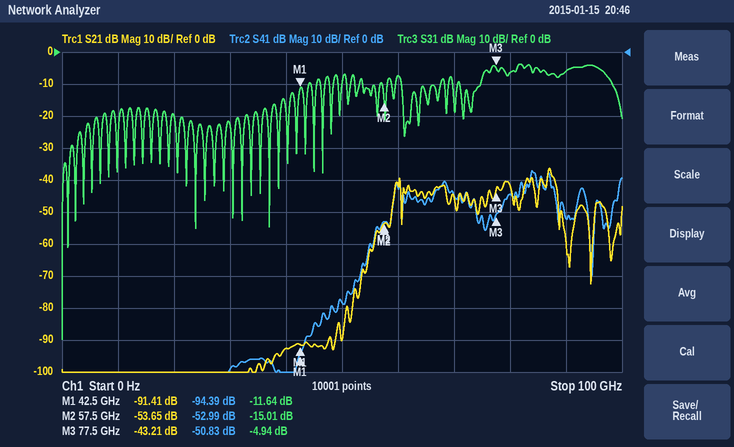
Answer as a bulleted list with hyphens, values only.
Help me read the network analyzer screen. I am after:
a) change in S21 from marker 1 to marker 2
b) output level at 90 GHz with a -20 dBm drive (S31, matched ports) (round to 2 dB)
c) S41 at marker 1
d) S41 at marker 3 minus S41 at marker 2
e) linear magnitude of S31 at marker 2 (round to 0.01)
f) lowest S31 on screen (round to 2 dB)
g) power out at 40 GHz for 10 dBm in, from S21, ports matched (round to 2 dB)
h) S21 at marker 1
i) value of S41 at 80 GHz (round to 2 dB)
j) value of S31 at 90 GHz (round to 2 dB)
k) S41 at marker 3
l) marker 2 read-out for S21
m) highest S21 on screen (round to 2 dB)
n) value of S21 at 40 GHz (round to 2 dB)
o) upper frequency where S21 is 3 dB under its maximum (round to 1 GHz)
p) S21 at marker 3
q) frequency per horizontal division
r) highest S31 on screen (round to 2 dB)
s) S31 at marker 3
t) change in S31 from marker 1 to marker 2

- 37.76 dB
- -26 dBm
- -94.39 dB
- 2.16 dB
- 0.18
- -90 dB
- -82 dBm
- -91.41 dB
- -44 dB
- -6 dB
- -50.83 dB
- -53.65 dB
- -36 dB
- -92 dB
- 88 GHz
- -43.21 dB
- 10 GHz
- -4 dB
- -4.94 dB
- -3.37 dB
